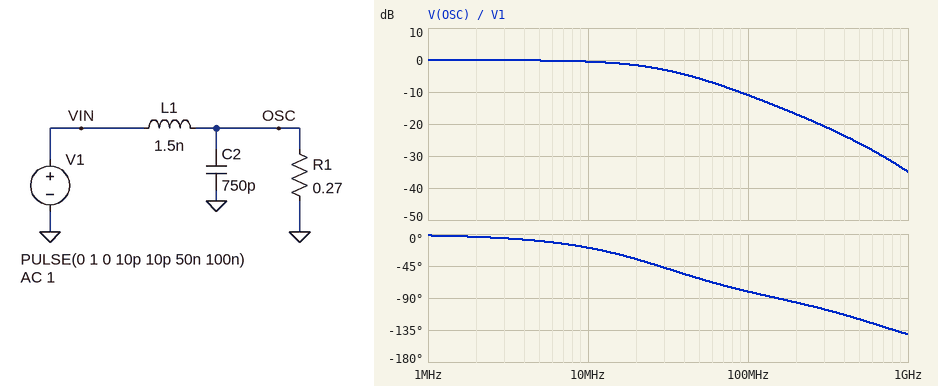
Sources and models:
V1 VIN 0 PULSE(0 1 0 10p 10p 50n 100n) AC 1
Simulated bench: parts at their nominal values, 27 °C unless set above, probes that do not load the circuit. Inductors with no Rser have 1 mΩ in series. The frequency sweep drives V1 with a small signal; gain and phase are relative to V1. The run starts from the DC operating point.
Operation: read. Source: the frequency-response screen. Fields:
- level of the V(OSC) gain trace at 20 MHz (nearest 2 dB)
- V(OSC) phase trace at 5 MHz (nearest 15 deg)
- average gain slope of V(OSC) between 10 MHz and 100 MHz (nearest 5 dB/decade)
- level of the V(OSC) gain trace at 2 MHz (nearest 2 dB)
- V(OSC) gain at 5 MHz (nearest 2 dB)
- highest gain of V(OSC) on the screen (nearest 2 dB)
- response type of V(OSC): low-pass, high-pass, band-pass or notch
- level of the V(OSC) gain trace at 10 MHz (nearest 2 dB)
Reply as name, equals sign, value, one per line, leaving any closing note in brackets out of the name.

level of the V(OSC) gain trace at 20 MHz = -2 dB
V(OSC) phase trace at 5 MHz = -15 deg
average gain slope of V(OSC) between 10 MHz and 100 MHz = -10 dB/decade
level of the V(OSC) gain trace at 2 MHz = 0 dB
V(OSC) gain at 5 MHz = 0 dB
highest gain of V(OSC) on the screen = 0 dB
response type of V(OSC): low-pass, high-pass, band-pass or notch = low-pass
level of the V(OSC) gain trace at 10 MHz = 0 dB
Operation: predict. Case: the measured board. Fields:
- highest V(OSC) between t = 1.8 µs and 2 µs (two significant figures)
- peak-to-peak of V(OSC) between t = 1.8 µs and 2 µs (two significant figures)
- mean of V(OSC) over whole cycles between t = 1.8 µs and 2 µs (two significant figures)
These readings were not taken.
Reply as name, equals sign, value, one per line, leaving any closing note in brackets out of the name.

highest V(OSC) between t = 1.8 µs and 2 µs = 1.0 V
peak-to-peak of V(OSC) between t = 1.8 µs and 2 µs = 1.0 V
mean of V(OSC) over whole cycles between t = 1.8 µs and 2 µs = 500 mV
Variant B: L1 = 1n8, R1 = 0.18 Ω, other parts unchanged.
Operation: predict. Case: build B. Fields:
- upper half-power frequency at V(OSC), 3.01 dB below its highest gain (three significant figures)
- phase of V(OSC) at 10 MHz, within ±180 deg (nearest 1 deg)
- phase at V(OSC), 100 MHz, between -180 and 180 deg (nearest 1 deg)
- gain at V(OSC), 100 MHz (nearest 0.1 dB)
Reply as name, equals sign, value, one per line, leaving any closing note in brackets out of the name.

upper half-power frequency at V(OSC), 3.01 dB below its highest gain = 16.2 MHz
phase of V(OSC) at 10 MHz, within ±180 deg = -32 deg
phase at V(OSC), 100 MHz, between -180 and 180 deg = -86 deg
gain at V(OSC), 100 MHz = -16.0 dB
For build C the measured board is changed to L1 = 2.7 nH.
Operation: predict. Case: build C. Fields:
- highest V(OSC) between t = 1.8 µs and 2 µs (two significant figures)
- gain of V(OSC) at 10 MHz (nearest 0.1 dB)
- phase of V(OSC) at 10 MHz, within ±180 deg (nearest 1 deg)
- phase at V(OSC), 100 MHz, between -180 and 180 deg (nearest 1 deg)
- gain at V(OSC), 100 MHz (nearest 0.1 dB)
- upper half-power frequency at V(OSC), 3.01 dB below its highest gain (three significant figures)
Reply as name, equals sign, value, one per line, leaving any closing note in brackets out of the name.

highest V(OSC) between t = 1.8 µs and 2 µs = 990 mV
gain of V(OSC) at 10 MHz = -1.4 dB
phase of V(OSC) at 10 MHz, within ±180 deg = -32 deg
phase at V(OSC), 100 MHz, between -180 and 180 deg = -88 deg
gain at V(OSC), 100 MHz = -16.0 dB
upper half-power frequency at V(OSC), 3.01 dB below its highest gain = 16.3 MHz
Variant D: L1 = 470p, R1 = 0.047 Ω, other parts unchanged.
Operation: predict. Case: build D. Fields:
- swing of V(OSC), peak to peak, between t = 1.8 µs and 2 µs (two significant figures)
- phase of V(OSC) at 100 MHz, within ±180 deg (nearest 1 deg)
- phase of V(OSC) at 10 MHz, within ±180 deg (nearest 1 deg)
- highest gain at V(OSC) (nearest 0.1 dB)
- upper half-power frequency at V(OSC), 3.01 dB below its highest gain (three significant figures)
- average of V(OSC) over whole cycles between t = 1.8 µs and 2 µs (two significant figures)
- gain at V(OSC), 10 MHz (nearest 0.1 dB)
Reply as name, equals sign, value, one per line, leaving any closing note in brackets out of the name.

swing of V(OSC), peak to peak, between t = 1.8 µs and 2 µs = 970 mV
phase of V(OSC) at 100 MHz, within ±180 deg = -82 deg
phase of V(OSC) at 10 MHz, within ±180 deg = -32 deg
highest gain at V(OSC) = -0.2 dB
upper half-power frequency at V(OSC), 3.01 dB below its highest gain = 16.3 MHz
average of V(OSC) over whole cycles between t = 1.8 µs and 2 µs = 490 mV
gain at V(OSC), 10 MHz = -1.6 dB
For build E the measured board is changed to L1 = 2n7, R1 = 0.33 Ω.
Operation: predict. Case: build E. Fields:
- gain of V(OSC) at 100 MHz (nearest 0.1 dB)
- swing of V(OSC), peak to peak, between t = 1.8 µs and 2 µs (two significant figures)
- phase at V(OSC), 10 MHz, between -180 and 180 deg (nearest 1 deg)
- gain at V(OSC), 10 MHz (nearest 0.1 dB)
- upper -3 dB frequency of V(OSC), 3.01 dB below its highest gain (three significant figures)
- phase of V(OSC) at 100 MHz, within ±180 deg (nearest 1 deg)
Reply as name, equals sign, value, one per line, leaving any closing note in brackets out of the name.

gain of V(OSC) at 100 MHz = -14.2 dB
swing of V(OSC), peak to peak, between t = 1.8 µs and 2 µs = 990 mV
phase at V(OSC), 10 MHz, between -180 and 180 deg = -27 deg
gain at V(OSC), 10 MHz = -1.0 dB
upper -3 dB frequency of V(OSC), 3.01 dB below its highest gain = 20.1 MHz
phase of V(OSC) at 100 MHz, within ±180 deg = -88 deg
